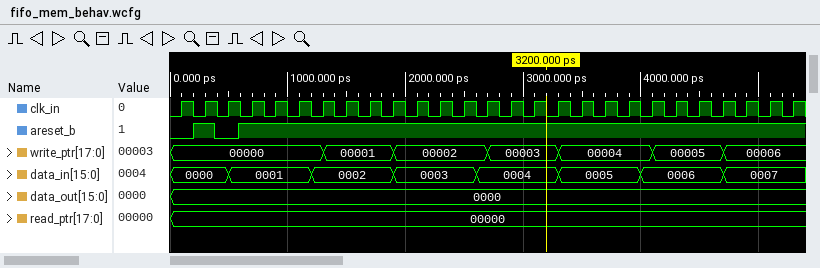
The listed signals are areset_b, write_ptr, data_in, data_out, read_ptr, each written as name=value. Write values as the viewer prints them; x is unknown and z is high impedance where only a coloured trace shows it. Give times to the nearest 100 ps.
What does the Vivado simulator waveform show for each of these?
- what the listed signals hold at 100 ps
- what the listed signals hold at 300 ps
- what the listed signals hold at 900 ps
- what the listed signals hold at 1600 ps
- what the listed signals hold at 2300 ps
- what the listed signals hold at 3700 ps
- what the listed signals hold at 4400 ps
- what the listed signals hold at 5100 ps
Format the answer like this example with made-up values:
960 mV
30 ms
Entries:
areset_b=0, write_ptr=00000, data_in=0000, data_out=0000, read_ptr=00000
areset_b=1, write_ptr=00000, data_in=0000, data_out=0000, read_ptr=00000
areset_b=1, write_ptr=00000, data_in=0001, data_out=0000, read_ptr=00000
areset_b=1, write_ptr=00001, data_in=0002, data_out=0000, read_ptr=00000
areset_b=1, write_ptr=00002, data_in=0003, data_out=0000, read_ptr=00000
areset_b=1, write_ptr=00004, data_in=0005, data_out=0000, read_ptr=00000
areset_b=1, write_ptr=00005, data_in=0006, data_out=0000, read_ptr=00000
areset_b=1, write_ptr=00006, data_in=0007, data_out=0000, read_ptr=00000
